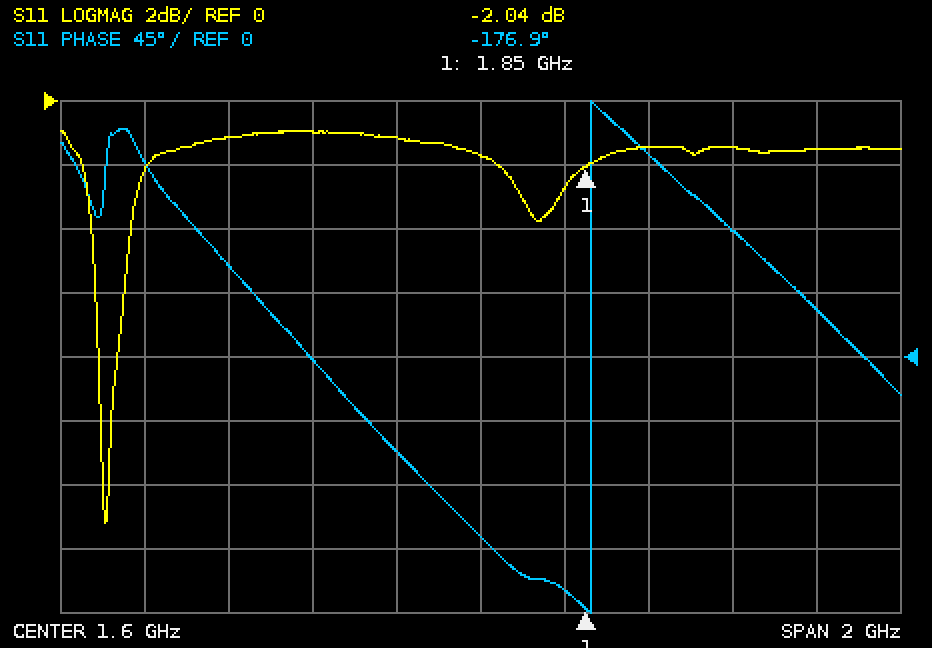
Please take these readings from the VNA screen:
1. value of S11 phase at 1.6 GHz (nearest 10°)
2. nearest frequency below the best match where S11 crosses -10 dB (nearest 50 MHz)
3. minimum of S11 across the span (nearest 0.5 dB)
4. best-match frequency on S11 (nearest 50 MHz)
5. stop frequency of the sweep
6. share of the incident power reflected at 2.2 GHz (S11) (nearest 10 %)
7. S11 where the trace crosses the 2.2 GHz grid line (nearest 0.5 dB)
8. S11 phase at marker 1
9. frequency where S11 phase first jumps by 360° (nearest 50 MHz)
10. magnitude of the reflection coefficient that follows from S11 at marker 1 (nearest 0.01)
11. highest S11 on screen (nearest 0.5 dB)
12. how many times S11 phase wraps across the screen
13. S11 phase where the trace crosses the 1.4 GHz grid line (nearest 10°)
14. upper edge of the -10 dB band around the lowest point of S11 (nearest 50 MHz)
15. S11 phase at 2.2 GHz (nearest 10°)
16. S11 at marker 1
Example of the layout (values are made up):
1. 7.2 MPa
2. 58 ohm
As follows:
1. -130°
2. 700 MHz
3. -13.0 dB
4. 700 MHz
5. 2.6 GHz
6. 70 %
7. -1.5 dB
8. -176.9°
9. 1.85 GHz
10. 0.79
11. -1.0 dB
12. 1
13. -70°
14. 700 MHz
15. 90°
16. -2.04 dB
